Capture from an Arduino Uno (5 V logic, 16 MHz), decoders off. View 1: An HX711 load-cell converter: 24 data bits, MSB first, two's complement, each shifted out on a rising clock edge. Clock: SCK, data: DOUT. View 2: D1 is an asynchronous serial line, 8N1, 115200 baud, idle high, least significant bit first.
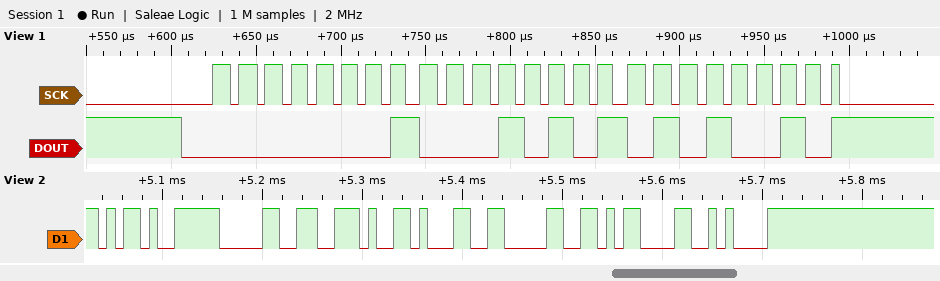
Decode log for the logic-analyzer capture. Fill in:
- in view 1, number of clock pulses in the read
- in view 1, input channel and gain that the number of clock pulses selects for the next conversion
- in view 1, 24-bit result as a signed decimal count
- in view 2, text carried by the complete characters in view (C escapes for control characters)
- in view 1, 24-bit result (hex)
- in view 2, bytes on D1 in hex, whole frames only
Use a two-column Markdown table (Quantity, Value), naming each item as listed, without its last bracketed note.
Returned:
| Quantity | Value |
|---|---|
| in view 1, number of clock pulses in the read | 25 |
| in view 1, input channel and gain that the number of clock pulses selects for the next conversion | channel A, gain 128 |
| in view 1, 24-bit result as a signed decimal count | 70994 |
| in view 2, text carried by the complete characters in view | "-0.10\r\n" |
| in view 1, 24-bit result | 0x011552 |
| in view 2, bytes on D1 in hex, whole frames only | 2D 30 2E 31 30 0D 0A |
